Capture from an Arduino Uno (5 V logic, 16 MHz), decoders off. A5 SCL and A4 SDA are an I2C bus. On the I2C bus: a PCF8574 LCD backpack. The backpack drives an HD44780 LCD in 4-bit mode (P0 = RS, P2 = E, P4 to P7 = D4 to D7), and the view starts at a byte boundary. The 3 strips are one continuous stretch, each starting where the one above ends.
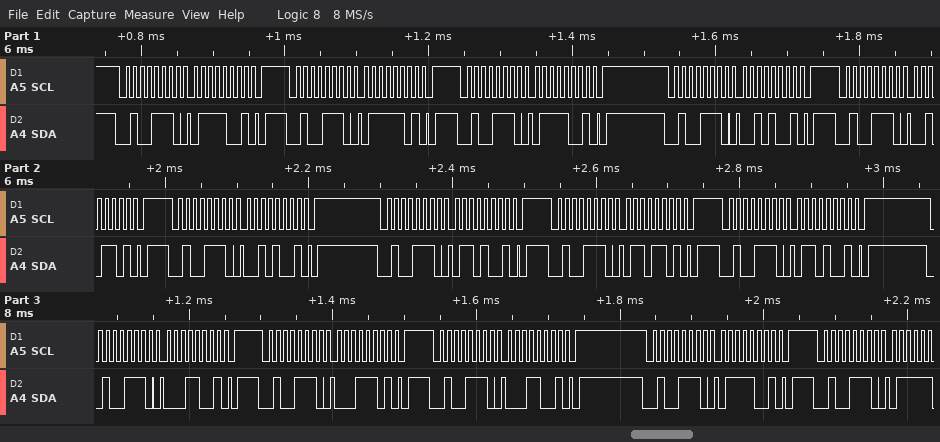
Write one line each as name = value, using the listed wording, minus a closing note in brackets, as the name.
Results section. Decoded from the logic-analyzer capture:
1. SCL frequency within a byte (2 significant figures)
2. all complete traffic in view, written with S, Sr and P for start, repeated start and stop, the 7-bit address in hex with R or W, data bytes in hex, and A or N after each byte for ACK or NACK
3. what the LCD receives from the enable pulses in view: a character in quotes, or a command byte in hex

SCL frequency within a byte = 100 kHz
all complete traffic in view, written with S, Sr and P for start, repeated start and stop, the 7-bit address in hex with R or W, data bytes in hex, and A or N after each byte for ACK or NACK = S 27W A 79 A P S 27W A 7D A P S 27W A 79 A P S 27W A 29 A P S 27W A 2D A P S 27W A 29 A P S 27W A 69 A P S 27W A 6D A P S 27W A 69 A P S 27W A 19 A P S 27W A 1D A P S 27W A 19 A P S 27W A 79 A P S 27W A
what the LCD receives from the enable pulses in view: a character in quotes, or a command byte in hex = 'r' 'a'
